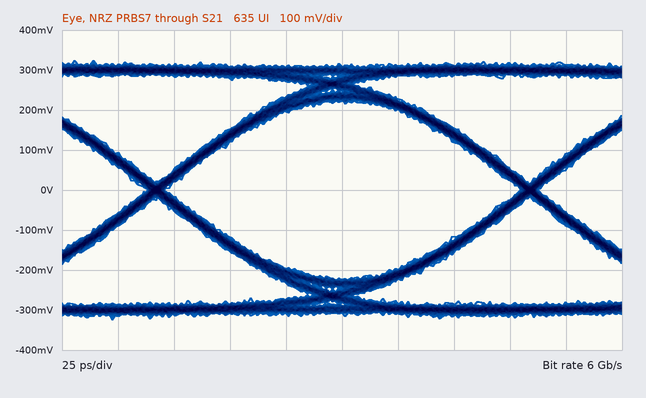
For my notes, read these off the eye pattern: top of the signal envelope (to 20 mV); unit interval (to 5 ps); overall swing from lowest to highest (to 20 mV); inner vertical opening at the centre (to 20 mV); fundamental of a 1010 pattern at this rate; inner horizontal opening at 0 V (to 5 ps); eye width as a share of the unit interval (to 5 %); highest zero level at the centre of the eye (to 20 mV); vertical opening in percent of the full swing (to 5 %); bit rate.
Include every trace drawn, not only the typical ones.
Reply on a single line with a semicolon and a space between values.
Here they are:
320 mV; 165 ps; 640 mV; 440 mV; 3 GHz; 160 ps; 95 %; -220 mV; 70 %; 6 Gb/s
